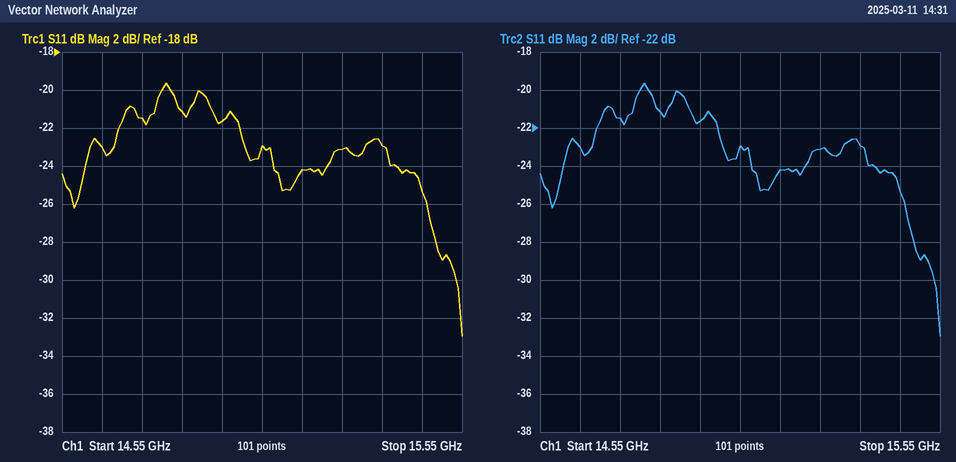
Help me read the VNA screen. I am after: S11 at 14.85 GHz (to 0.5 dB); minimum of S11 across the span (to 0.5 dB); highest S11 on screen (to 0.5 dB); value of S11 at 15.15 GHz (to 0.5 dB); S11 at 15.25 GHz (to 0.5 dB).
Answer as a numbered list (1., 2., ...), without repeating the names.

1. -21.0 dB
2. -33.0 dB
3. -19.5 dB
4. -24.0 dB
5. -23.0 dB
